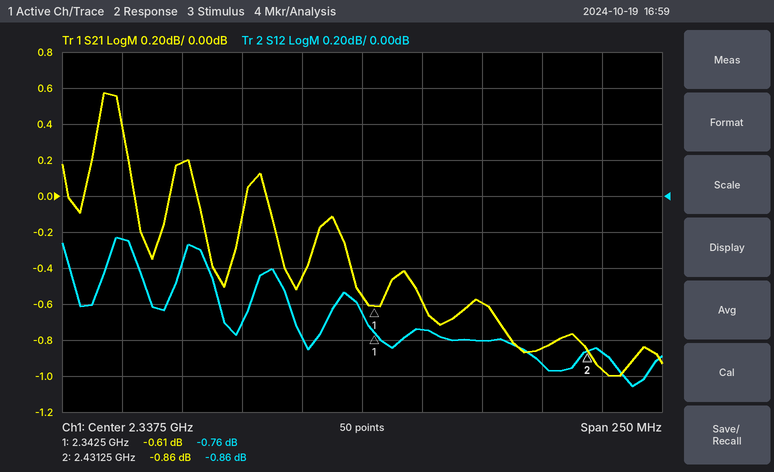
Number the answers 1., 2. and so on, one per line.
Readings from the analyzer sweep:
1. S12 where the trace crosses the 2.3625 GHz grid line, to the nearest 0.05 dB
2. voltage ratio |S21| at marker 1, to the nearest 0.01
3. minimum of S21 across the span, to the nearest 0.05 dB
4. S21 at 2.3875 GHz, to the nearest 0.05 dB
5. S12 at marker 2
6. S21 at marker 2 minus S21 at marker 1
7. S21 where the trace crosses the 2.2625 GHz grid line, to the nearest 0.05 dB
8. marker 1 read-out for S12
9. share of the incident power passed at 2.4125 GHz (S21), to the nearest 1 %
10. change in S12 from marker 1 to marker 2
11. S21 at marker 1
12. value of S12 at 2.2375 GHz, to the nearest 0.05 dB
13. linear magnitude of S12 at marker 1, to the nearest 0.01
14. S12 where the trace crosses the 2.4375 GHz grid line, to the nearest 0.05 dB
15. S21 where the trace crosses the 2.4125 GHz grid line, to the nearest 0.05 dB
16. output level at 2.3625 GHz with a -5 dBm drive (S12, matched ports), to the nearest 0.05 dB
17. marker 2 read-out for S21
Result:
1. -0.75 dB
2. 0.93
3. -1.00 dB
4. -0.60 dB
5. -0.86 dB
6. -0.25 dB
7. 0.20 dB
8. -0.76 dB
9. 82 %
10. -0.10 dB
11. -0.61 dB
12. -0.25 dB
13. 0.92
14. -0.85 dB
15. -0.85 dB
16. -5.75 dBm
17. -0.86 dB
